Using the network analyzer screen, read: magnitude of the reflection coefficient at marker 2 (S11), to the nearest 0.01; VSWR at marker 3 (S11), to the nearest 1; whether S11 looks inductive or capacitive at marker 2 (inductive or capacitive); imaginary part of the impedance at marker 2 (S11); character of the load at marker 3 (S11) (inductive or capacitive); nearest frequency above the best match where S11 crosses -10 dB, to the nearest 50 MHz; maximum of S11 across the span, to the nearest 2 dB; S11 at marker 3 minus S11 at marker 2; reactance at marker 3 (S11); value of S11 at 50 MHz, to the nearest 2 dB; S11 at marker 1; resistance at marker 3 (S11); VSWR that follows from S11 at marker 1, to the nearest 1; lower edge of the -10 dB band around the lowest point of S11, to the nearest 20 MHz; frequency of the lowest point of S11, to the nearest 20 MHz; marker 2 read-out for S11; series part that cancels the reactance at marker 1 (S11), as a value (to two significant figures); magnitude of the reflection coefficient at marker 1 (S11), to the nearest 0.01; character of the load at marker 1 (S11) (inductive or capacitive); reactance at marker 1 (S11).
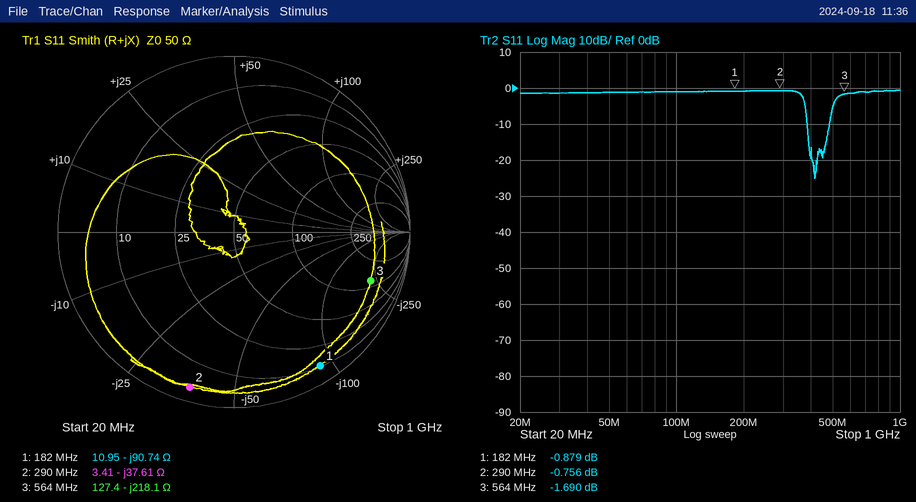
0.92
10
capacitive
-37.61 Ω
capacitive
500 MHz
0 dB
-0.934 dB
-218.1 Ω
-2 dB
-0.879 dB
127.4 Ω
20
380 MHz
420 MHz
-0.756 dB
79 nH
0.90
capacitive
-90.74 Ω
